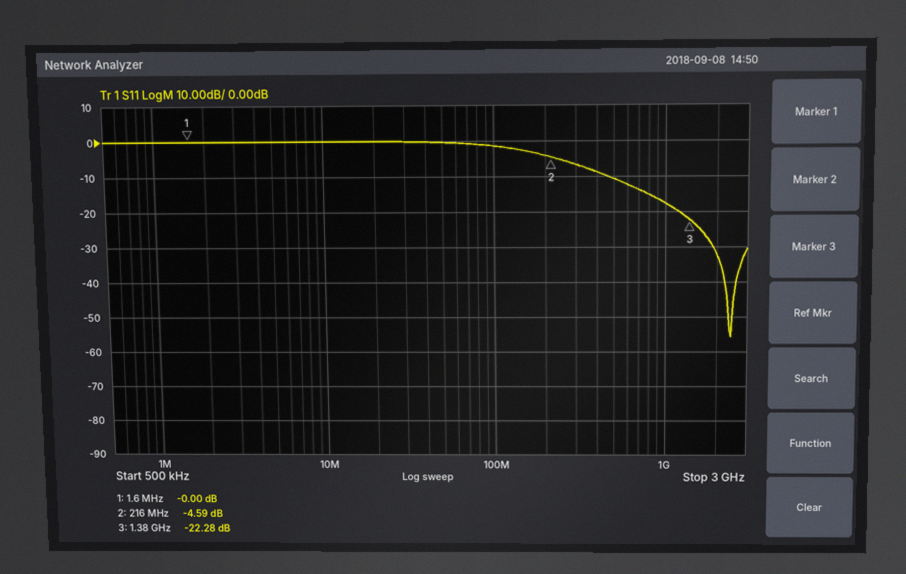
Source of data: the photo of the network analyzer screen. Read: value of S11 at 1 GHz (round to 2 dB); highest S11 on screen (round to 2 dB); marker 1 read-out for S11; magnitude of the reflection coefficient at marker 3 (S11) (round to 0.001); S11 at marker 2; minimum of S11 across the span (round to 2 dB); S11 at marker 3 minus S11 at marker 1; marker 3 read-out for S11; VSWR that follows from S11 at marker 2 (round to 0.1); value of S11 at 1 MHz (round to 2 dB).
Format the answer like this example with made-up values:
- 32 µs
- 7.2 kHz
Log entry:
- -18 dB
- 0 dB
- -0.00 dB
- 0.077
- -4.59 dB
- -56 dB
- -22.28 dB
- -22.28 dB
- 3.9
- 0 dB
